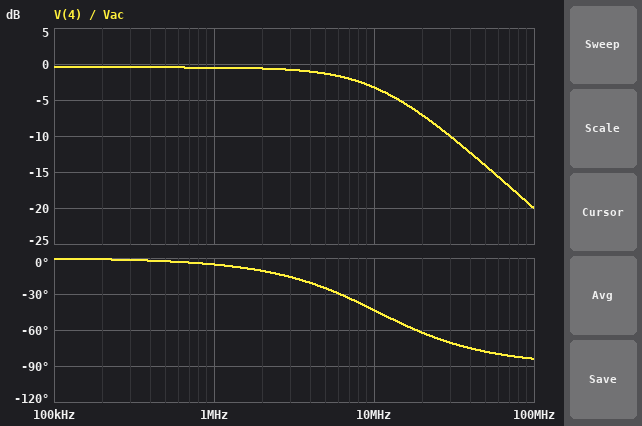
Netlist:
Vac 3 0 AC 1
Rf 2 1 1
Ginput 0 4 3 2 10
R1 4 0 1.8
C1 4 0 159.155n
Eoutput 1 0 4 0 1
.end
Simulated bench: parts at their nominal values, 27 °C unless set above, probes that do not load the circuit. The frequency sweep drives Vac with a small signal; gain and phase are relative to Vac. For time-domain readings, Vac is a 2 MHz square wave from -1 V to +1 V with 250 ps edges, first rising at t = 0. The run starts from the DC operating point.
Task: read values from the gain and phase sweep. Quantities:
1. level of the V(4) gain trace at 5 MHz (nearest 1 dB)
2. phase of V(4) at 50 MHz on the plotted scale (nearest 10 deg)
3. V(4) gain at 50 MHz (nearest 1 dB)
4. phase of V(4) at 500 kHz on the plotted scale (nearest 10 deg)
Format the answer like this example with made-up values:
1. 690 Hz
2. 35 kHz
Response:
1. -1 dB
2. -80 deg
3. -14 dB
4. 0 deg
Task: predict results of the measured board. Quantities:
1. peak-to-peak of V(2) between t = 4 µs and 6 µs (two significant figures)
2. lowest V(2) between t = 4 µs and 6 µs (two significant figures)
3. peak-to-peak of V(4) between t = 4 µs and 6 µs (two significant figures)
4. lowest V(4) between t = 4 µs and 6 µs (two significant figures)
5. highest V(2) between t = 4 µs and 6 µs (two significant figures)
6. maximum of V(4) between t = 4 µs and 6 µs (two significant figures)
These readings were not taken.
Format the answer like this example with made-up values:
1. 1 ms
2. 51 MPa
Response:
1. 1.9 V
2. -950 mV
3. 1.9 V
4. -950 mV
5. 950 mV
6. 950 mV
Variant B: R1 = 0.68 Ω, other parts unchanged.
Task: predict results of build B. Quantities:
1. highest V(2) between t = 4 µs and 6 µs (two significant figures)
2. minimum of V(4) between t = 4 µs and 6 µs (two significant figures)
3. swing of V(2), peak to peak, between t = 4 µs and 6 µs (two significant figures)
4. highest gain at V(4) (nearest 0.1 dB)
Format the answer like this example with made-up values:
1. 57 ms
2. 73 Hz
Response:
1. 870 mV
2. -870 mV
3. 1.7 V
4. -1.2 dB
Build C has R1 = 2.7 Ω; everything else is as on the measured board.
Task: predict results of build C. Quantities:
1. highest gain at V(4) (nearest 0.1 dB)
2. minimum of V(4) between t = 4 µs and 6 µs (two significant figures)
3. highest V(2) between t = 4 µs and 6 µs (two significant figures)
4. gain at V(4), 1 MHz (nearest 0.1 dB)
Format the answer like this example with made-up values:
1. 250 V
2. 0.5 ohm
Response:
1. -0.3 dB
2. -960 mV
3. 960 mV
4. -0.4 dB
